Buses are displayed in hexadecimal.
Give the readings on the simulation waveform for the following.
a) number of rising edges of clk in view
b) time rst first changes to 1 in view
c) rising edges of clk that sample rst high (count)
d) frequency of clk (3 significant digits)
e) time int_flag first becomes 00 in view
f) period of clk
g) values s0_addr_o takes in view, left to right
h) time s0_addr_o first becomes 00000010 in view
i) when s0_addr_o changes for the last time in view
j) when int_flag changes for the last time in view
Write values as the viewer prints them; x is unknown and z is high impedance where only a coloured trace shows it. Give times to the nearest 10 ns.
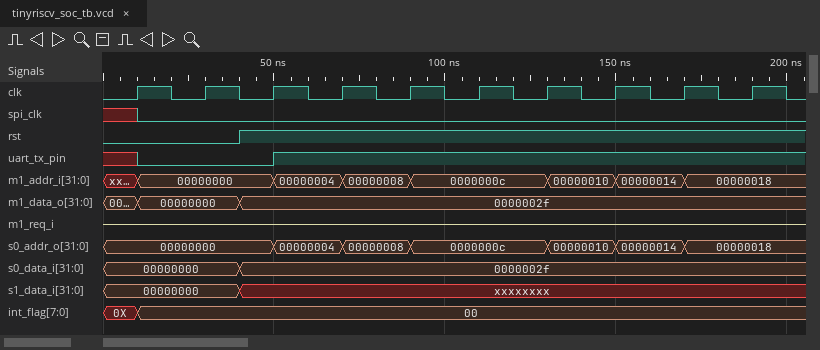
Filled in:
10
40 ns
8
50.0 MHz
10 ns
20 ns
00000000, 00000004, 00000008, 0000000c, 00000010, 00000014, 00000018
130 ns
170 ns
10 ns
